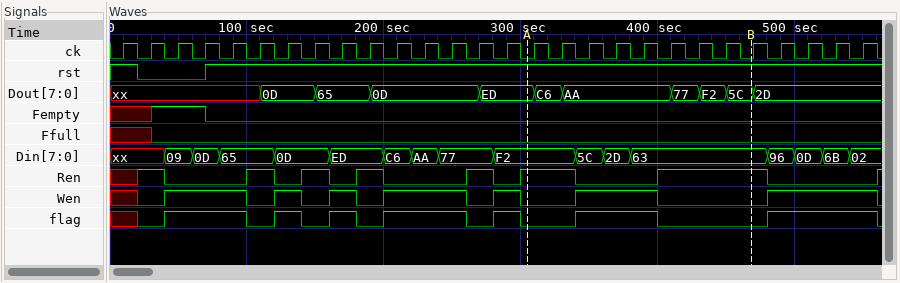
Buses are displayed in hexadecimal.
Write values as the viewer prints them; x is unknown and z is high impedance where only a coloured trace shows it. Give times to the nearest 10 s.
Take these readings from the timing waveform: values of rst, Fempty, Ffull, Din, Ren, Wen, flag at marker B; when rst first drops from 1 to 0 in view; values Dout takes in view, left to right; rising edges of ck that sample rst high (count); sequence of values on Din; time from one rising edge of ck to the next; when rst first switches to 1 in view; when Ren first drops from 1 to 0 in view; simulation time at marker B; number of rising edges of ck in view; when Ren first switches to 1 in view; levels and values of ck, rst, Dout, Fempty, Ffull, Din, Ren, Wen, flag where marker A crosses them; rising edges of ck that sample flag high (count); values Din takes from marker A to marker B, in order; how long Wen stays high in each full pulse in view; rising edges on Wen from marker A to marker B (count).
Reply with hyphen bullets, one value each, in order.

- rst=1, Fempty=0, Ffull=0, Din=63, Ren=1, Wen=0, flag=0
- 20 s
- xx, 0D, 65, 0D, ED, C6, AA, 77, F2, 5C, 2D
- 25
- xx, 09, 0D, 65, 0D, ED, C6, AA, 77, F2, 5C, 2D, 63, 96, 0D, 6B, 02
- 20 s
- 70 s
- 40 s
- 470 s
- 28
- 20 s
- ck=0, rst=1, Dout=ED, Fempty=0, Ffull=0, Din=F2, Ren=1, Wen=0, flag=0
- 16
- F2, 5C, 2D, 63
- 60 s, 20 s, 20 s, 60 s, 20 s, 60 s, 80 s
- 1
